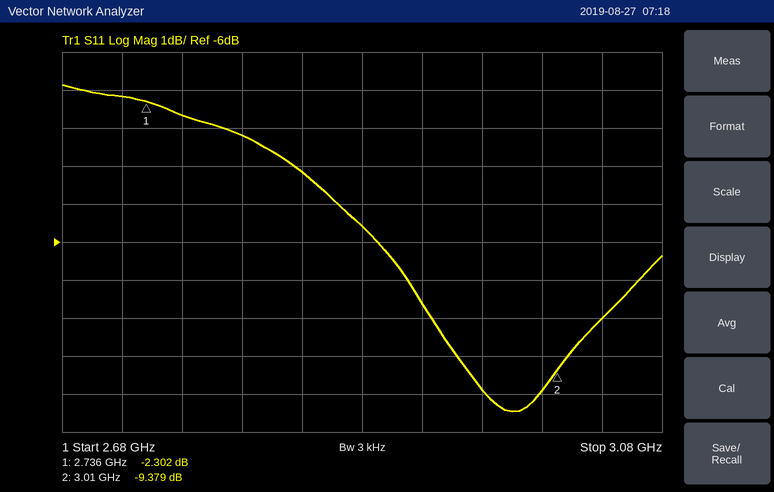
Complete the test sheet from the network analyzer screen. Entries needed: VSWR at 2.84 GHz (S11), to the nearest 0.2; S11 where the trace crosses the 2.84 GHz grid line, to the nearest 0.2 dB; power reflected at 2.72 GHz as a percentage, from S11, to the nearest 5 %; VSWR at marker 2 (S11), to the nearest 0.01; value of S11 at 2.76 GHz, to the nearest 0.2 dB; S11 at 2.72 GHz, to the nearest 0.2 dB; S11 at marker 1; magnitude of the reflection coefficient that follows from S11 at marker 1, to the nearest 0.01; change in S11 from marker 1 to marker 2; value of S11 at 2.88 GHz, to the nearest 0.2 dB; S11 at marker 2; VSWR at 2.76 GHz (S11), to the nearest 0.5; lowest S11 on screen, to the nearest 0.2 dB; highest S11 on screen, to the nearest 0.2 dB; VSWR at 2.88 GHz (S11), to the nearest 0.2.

4.2
-4.2 dB
60 %
2.03
-2.6 dB
-2.2 dB
-2.302 dB
0.77
-7.077 dB
-5.6 dB
-9.379 dB
6.5
-10.4 dB
-1.8 dB
3.2
